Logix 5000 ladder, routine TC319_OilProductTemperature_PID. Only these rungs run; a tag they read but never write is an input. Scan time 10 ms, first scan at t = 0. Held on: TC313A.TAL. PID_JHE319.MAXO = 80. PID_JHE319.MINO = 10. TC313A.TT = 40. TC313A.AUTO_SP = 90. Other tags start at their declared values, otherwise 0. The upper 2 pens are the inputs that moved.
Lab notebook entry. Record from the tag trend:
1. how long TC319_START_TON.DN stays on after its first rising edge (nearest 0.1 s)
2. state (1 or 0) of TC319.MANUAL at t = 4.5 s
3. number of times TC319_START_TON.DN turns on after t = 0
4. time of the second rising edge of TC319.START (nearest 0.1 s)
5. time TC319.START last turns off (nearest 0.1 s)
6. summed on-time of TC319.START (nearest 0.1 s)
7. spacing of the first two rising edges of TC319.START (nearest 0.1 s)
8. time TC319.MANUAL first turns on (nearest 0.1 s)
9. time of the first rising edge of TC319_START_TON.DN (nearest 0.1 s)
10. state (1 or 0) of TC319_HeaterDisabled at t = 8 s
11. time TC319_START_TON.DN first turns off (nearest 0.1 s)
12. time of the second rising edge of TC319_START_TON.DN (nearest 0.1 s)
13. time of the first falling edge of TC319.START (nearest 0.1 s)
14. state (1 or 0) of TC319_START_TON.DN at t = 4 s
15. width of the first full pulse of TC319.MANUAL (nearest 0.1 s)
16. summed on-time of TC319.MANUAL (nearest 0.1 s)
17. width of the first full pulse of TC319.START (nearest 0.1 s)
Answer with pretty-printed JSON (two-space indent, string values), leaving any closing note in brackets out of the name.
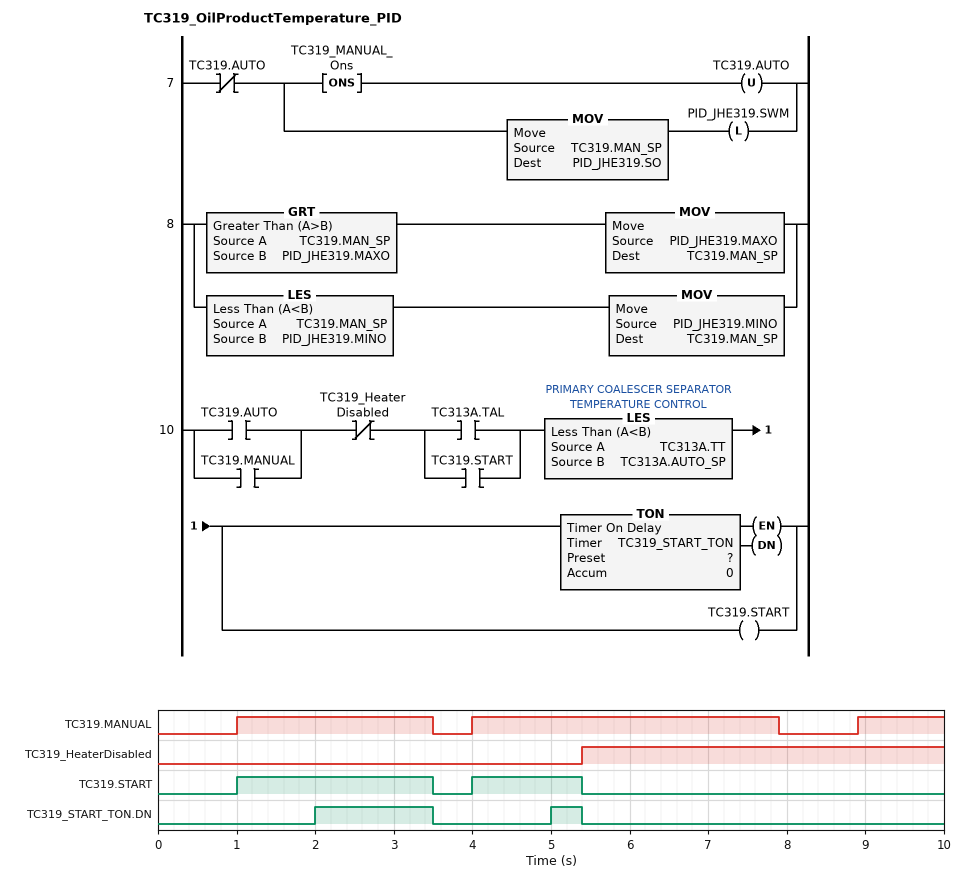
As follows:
{
  "how long TC319_START_TON.DN stays on after its first rising edge": "1.5 s",
  "state (1 or 0) of TC319.MANUAL at t = 4.5 s": "1",
  "number of times TC319_START_TON.DN turns on after t = 0": "2",
  "time of the second rising edge of TC319.START": "4.0 s",
  "time TC319.START last turns off": "5.4 s",
  "summed on-time of TC319.START": "3.9 s",
  "spacing of the first two rising edges of TC319.START": "3.0 s",
  "time TC319.MANUAL first turns on": "1.0 s",
  "time of the first rising edge of TC319_START_TON.DN": "2.0 s",
  "state (1 or 0) of TC319_HeaterDisabled at t = 8 s": "1",
  "time TC319_START_TON.DN first turns off": "3.5 s",
  "time of the second rising edge of TC319_START_TON.DN": "5.0 s",
  "time of the first falling edge of TC319.START": "3.5 s",
  "state (1 or 0) of TC319_START_TON.DN at t = 4 s": "0",
  "width of the first full pulse of TC319.MANUAL": "2.5 s",
  "summed on-time of TC319.MANUAL": "7.5 s",
  "width of the first full pulse of TC319.START": "2.5 s"
}
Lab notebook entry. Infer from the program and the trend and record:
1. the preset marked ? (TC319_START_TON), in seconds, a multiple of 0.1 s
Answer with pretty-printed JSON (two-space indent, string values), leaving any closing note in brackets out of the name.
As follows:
{
  "the preset marked ? (TC319_START_TON), in seconds, a multiple of 0.1 s": "1.0 s"
}
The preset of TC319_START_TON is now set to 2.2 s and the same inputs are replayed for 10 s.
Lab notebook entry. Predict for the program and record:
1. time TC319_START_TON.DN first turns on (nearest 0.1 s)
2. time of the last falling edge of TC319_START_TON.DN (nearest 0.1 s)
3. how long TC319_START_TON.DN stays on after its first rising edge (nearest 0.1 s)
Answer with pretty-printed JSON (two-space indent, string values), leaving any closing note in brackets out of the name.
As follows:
{
  "time TC319_START_TON.DN first turns on": "3.2 s",
  "time of the last falling edge of TC319_START_TON.DN": "3.5 s",
  "how long TC319_START_TON.DN stays on after its first rising edge": "0.3 s"
}
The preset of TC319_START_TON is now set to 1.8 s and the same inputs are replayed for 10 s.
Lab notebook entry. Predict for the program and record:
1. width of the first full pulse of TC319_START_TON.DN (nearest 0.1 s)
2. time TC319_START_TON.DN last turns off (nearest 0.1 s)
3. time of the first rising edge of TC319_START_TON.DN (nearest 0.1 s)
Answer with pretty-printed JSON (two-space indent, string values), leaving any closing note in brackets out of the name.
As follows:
{
  "width of the first full pulse of TC319_START_TON.DN": "0.7 s",
  "time TC319_START_TON.DN last turns off": "3.5 s",
  "time of the first rising edge of TC319_START_TON.DN": "2.8 s"
}
